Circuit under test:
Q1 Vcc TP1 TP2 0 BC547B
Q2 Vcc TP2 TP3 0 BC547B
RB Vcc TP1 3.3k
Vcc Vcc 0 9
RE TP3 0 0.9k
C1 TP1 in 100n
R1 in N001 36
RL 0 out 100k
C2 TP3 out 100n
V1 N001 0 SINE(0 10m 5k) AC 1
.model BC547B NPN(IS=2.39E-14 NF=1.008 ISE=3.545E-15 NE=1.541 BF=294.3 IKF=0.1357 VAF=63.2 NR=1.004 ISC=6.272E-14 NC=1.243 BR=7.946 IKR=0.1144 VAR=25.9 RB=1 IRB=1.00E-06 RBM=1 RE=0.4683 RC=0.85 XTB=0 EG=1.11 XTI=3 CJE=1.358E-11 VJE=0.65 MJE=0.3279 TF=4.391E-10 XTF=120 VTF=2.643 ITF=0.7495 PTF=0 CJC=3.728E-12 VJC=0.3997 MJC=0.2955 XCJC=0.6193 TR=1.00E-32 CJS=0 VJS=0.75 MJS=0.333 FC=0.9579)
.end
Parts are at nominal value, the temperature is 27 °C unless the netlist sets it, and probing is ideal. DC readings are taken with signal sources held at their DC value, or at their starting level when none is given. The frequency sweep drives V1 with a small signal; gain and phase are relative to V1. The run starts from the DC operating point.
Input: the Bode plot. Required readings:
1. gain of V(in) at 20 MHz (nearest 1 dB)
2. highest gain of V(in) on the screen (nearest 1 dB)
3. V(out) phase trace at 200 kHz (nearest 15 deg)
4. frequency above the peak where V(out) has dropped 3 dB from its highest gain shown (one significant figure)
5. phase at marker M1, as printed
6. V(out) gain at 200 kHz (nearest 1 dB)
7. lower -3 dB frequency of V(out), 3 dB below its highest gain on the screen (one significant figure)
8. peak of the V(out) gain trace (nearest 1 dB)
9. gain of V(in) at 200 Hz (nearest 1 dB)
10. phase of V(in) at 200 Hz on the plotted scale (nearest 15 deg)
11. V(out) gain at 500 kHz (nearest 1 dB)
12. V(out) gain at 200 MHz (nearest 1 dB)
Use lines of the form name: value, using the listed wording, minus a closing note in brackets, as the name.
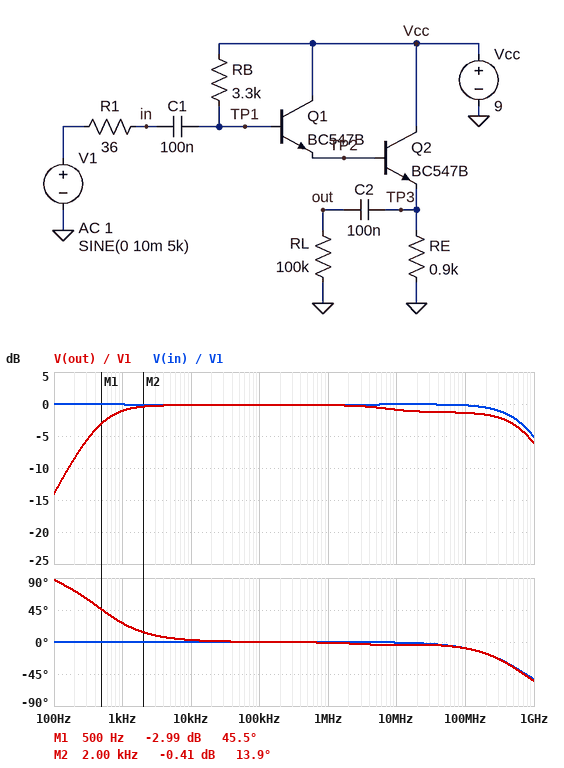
gain of V(in) at 20 MHz: 0 dB
highest gain of V(in) on the screen: 0 dB
V(out) phase trace at 200 kHz: 0 deg
frequency above the peak where V(out) has dropped 3 dB from its highest gain shown: 500 MHz
phase at marker M1, as printed: 45.5 deg
V(out) gain at 200 kHz: 0 dB
lower -3 dB frequency of V(out), 3 dB below its highest gain on the screen: 500 Hz
peak of the V(out) gain trace: 0 dB
gain of V(in) at 200 Hz: 0 dB
phase of V(in) at 200 Hz on the plotted scale: 0 deg
V(out) gain at 500 kHz: 0 dB
V(out) gain at 200 MHz: -2 dB
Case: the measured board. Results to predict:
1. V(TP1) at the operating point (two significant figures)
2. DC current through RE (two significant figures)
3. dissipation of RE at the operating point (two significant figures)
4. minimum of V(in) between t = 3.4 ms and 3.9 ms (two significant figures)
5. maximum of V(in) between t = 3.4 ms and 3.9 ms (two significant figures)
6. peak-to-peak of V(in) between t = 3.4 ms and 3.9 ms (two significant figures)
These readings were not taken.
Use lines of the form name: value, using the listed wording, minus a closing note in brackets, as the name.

V(TP1) at the operating point: 9.0 V
DC current through RE: 8.6 mA
dissipation of RE at the operating point: 67 mW
minimum of V(in) between t = 3.4 ms and 3.9 ms: -9.9 mV
maximum of V(in) between t = 3.4 ms and 3.9 ms: 9.9 mV
peak-to-peak of V(in) between t = 3.4 ms and 3.9 ms: 20 mV
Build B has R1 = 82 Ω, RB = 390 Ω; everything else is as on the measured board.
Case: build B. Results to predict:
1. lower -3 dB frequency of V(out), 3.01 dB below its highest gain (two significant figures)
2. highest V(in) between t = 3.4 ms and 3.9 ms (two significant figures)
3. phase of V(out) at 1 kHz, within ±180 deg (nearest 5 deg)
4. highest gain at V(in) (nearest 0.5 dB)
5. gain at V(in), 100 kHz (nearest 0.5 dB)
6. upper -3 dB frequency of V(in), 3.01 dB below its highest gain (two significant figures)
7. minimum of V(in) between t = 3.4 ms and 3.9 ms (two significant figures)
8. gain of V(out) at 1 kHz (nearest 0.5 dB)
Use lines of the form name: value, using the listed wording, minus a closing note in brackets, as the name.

lower -3 dB frequency of V(out), 3.01 dB below its highest gain: 3.4 kHz
highest V(in) between t = 3.4 ms and 3.9 ms: 8.8 mV
phase of V(out) at 1 kHz, within ±180 deg: 75 deg
highest gain at V(in): 0 dB
gain at V(in), 100 kHz: -1.5 dB
upper -3 dB frequency of V(in), 3.01 dB below its highest gain: 200 MHz
minimum of V(in) between t = 3.4 ms and 3.9 ms: -8.8 mV
gain of V(out) at 1 kHz: -12.5 dB
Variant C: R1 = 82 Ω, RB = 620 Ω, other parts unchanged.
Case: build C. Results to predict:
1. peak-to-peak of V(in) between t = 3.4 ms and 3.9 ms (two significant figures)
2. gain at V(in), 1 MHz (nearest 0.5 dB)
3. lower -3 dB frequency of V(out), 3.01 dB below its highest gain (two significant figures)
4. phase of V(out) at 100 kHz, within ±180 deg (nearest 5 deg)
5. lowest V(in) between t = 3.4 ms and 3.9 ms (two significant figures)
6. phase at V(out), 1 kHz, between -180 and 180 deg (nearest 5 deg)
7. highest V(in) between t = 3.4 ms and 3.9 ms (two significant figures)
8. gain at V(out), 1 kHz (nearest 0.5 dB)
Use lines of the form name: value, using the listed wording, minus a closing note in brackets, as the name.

peak-to-peak of V(in) between t = 3.4 ms and 3.9 ms: 18 mV
gain at V(in), 1 MHz: -1.0 dB
lower -3 dB frequency of V(out), 3.01 dB below its highest gain: 2.3 kHz
phase of V(out) at 100 kHz, within ±180 deg: 0 deg
lowest V(in) between t = 3.4 ms and 3.9 ms: -9.0 mV
phase at V(out), 1 kHz, between -180 and 180 deg: 65 deg
highest V(in) between t = 3.4 ms and 3.9 ms: 9.0 mV
gain at V(out), 1 kHz: -9.0 dB
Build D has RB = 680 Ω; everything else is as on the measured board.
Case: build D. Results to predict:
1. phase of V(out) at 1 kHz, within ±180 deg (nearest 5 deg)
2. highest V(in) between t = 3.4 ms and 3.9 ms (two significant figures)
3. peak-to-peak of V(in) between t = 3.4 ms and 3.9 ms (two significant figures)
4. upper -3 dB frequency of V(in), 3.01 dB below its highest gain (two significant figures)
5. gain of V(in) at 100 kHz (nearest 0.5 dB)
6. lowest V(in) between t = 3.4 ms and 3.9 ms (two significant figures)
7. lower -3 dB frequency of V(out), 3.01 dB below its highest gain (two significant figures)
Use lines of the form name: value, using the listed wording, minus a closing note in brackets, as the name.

phase of V(out) at 1 kHz, within ±180 deg: 65 deg
highest V(in) between t = 3.4 ms and 3.9 ms: 9.6 mV
peak-to-peak of V(in) between t = 3.4 ms and 3.9 ms: 19 mV
upper -3 dB frequency of V(in), 3.01 dB below its highest gain: 610 MHz
gain of V(in) at 100 kHz: -0.5 dB
lowest V(in) between t = 3.4 ms and 3.9 ms: -9.6 mV
lower -3 dB frequency of V(out), 3.01 dB below its highest gain: 2.2 kHz
